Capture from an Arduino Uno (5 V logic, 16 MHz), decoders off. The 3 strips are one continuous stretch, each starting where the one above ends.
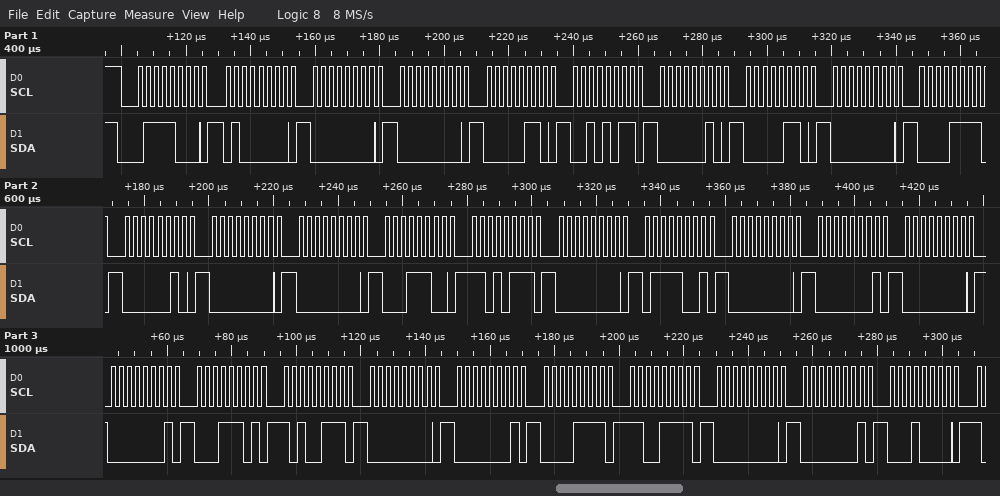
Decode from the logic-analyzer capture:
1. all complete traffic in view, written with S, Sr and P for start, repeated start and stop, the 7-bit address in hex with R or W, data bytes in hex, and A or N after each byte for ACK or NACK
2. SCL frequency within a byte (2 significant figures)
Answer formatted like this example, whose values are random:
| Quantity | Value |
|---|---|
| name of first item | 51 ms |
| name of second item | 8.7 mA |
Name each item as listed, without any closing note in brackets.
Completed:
| Quantity | Value |
|---|---|
| all complete traffic in view, written with S, Sr and P for start, repeated start and stop, the 7-bit address in hex with R or W, data bytes in hex, and A or N after each byte for ACK or NACK | S 3CW A 40 A 00 A 00 A 06 A 2B A 02 A 06 A 00 A 0F A 02 A 00 A 00 A 1C A D7 A 00 A 79 A 00 A 01 A 00 A 01 A 1D A A7 A 00 A 01 A 0F A CF A 00 A 01 A 10 A |
| SCL frequency within a byte | 400 kHz |
